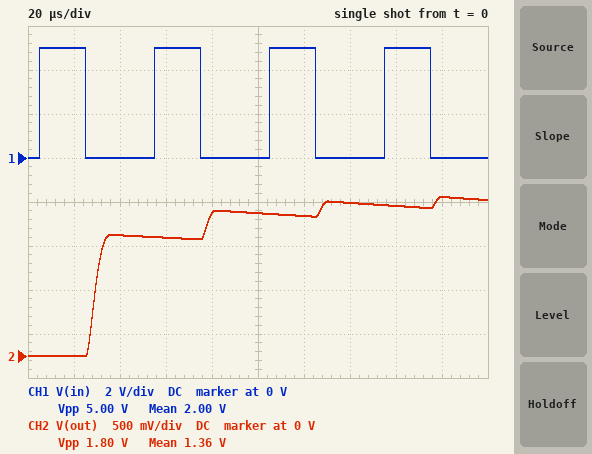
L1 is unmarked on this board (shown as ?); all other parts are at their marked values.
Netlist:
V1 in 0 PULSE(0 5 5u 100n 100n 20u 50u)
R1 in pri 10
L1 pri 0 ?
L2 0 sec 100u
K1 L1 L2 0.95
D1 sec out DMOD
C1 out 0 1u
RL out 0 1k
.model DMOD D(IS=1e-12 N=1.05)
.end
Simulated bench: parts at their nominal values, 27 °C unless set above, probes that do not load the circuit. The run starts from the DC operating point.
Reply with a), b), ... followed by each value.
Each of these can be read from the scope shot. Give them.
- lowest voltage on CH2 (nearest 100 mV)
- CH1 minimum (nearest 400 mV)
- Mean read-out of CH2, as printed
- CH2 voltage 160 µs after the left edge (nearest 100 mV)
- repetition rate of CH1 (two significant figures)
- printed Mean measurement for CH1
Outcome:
a) 0 V
b) 0 V
c) 1.36 V
d) 1.7 V
e) 20 kHz
f) 2.00 V
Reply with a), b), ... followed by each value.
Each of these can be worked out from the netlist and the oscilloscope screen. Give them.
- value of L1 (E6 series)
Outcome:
a) 150 µH
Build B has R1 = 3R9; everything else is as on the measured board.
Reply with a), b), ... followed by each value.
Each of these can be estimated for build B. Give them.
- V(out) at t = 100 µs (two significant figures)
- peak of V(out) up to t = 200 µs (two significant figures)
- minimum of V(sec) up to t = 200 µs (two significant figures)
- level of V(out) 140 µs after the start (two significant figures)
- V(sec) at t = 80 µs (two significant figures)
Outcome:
a) 1.2 V
b) 1.4 V
c) -3.9 V
d) 1.3 V
e) 1.8 V
